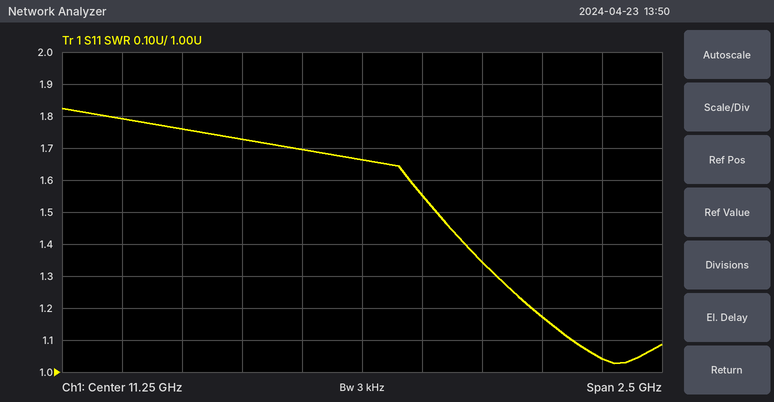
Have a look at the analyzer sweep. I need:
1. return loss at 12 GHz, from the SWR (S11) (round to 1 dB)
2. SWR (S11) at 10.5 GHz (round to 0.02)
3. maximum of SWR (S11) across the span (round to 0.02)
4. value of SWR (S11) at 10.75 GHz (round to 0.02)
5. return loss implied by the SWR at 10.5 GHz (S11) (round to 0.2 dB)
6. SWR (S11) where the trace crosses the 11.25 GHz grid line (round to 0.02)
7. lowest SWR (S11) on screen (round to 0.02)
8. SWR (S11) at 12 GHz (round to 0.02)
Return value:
22 dB
1.76
1.82
1.72
11.2 dB
1.66
1.02
1.18
